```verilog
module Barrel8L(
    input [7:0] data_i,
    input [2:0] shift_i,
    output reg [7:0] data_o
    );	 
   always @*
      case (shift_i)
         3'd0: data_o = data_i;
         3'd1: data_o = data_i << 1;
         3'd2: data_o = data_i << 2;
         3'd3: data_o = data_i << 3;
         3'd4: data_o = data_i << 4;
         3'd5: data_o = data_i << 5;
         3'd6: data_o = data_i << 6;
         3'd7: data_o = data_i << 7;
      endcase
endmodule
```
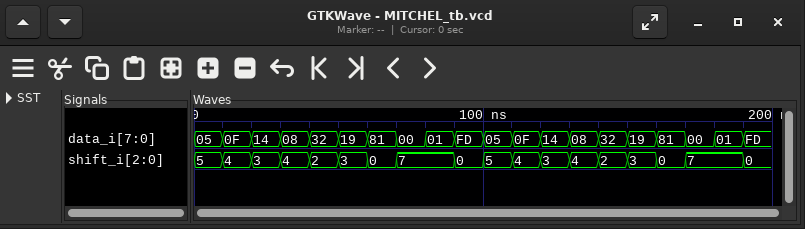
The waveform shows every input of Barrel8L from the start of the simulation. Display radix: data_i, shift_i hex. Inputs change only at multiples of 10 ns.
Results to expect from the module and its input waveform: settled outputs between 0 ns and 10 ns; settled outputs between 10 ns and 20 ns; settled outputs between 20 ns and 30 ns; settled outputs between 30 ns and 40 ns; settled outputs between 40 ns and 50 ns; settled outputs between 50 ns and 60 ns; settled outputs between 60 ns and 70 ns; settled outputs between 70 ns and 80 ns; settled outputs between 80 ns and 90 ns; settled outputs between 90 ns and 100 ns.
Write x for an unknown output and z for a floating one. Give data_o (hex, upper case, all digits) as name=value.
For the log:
data_o=A0
data_o=F0
data_o=A0
data_o=80
data_o=C8
data_o=C8
data_o=81
data_o=00
data_o=80
data_o=FD
